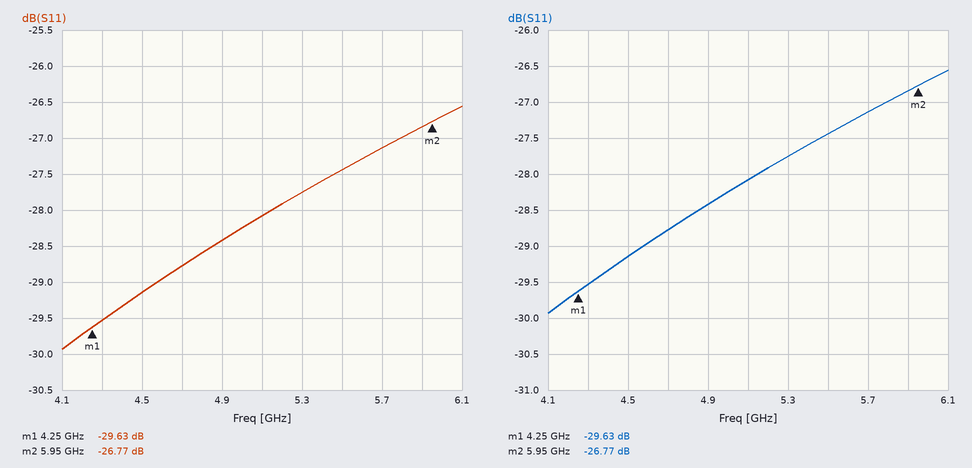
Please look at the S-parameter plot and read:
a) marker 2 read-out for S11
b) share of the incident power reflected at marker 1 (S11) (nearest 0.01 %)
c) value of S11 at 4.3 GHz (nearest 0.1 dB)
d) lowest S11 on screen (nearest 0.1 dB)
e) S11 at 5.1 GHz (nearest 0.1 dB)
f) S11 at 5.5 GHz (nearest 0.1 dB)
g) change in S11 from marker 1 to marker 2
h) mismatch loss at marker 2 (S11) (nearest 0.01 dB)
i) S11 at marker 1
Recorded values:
-26.77 dB
0.11 %
-29.5 dB
-29.9 dB
-28.1 dB
-27.4 dB
2.86 dB
0.01 dB
-29.63 dB
